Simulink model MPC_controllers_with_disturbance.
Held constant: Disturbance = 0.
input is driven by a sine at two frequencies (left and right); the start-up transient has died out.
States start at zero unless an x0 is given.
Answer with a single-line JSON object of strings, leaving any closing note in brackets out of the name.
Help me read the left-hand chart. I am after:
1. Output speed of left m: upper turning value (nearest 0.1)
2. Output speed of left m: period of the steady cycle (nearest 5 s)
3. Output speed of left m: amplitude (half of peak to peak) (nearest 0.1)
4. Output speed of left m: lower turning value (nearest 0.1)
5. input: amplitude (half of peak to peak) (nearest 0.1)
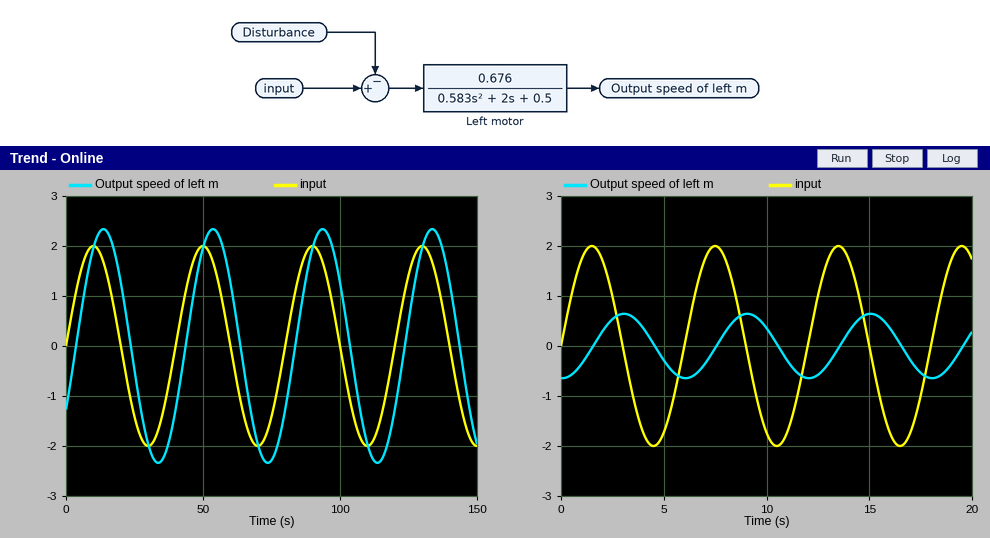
{"Output speed of left m: upper turning value": "2.3", "Output speed of left m: period of the steady cycle": "40 s", "Output speed of left m: amplitude (half of peak to peak)": "2.3", "Output speed of left m: lower turning value": "-2.3", "input: amplitude (half of peak to peak)": "2.0"}
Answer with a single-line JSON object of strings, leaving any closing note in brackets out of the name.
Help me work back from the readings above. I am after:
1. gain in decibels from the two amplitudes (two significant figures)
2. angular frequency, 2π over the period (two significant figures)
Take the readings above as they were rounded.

{"gain in decibels from the two amplitudes": "1.2 dB", "angular frequency, 2π over the period": "0.16 rad/s"}
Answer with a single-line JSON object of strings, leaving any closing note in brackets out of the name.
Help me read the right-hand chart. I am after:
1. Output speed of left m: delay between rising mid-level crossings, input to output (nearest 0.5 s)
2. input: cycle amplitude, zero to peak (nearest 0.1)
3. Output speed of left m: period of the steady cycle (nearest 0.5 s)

{"Output speed of left m: delay between rising mid-level crossings, input to output": "1.5 s", "input: cycle amplitude, zero to peak": "2.0", "Output speed of left m: period of the steady cycle": "6.0 s"}
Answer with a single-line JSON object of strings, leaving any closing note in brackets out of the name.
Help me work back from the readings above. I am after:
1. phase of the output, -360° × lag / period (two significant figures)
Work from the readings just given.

{"phase of the output, -360° × lag / period": "-90°"}
